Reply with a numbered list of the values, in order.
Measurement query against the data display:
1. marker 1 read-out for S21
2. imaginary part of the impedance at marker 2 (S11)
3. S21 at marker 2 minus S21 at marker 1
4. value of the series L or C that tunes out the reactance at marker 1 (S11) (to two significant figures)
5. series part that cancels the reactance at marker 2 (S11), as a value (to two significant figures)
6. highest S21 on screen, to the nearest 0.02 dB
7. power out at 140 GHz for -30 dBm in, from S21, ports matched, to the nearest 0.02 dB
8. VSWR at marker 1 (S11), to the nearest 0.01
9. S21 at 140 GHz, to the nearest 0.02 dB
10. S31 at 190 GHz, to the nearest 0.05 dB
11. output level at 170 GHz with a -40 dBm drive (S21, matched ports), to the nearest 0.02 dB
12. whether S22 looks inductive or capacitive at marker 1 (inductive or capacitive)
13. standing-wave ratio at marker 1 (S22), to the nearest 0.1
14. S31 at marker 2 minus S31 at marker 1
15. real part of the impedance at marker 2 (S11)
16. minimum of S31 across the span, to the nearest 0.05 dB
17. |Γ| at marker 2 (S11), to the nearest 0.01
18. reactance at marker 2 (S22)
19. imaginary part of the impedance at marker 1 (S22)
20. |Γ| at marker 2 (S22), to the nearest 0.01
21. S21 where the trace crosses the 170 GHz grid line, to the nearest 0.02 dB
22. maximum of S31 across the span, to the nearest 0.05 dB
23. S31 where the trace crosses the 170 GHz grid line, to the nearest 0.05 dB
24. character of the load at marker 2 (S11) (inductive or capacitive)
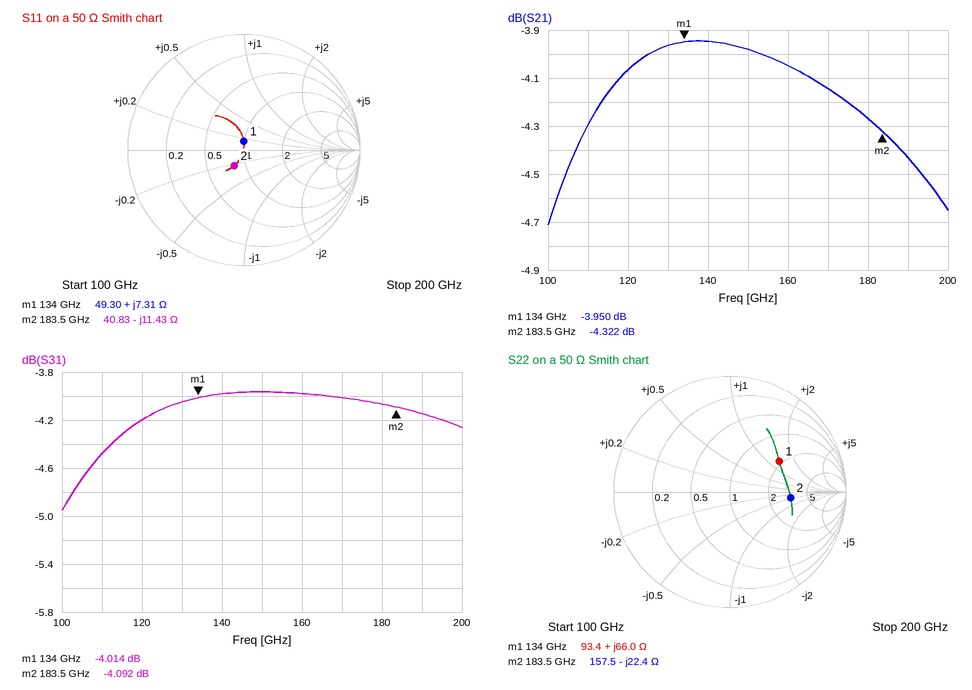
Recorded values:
1. -3.950 dB
2. -11.43 Ω
3. -0.372 dB
4. 160 fF
5. 9.9 pH
6. -3.94 dB
7. -33.94 dBm
8. 1.16
9. -3.94 dB
10. -4.15 dB
11. -44.14 dBm
12. inductive
13. 3.0
14. -0.078 dB
15. 40.83 Ω
16. -4.95 dB
17. 0.16
18. -22.4 Ω
19. +66.0 Ω
20. 0.53
21. -4.14 dB
22. -3.95 dB
23. -4.00 dB
24. capacitive
